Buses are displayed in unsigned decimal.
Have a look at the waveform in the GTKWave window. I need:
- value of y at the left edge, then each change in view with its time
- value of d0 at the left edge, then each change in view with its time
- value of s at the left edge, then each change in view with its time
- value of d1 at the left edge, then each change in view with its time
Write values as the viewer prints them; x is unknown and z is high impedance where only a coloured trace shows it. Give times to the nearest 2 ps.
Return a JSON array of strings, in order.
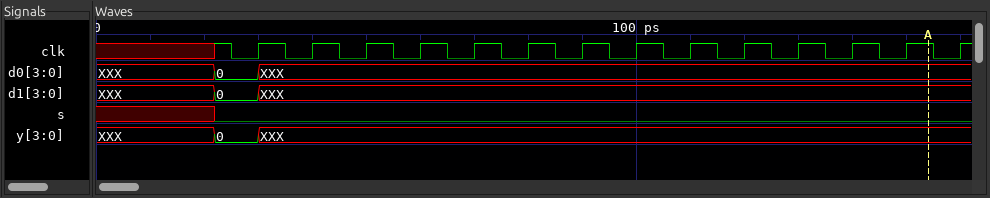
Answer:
["XXX, 0 at 22 ps, XXX at 30 ps", "XXX, 0 at 22 ps, XXX at 30 ps", "x, 0 at 22 ps", "XXX, 0 at 22 ps, XXX at 30 ps"]
